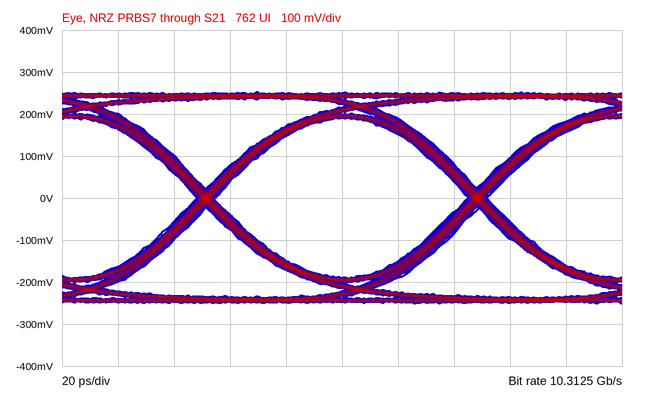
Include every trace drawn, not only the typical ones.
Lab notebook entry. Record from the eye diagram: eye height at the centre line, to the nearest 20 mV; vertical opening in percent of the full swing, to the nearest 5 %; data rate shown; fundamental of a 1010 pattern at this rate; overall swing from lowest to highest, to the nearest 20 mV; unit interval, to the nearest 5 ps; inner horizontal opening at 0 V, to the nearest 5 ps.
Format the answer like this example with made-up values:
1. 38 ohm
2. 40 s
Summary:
1. 380 mV
2. 75 %
3. 10.3125 Gb/s
4. 5.15625 GHz
5. 500 mV
6. 95 ps
7. 90 ps
